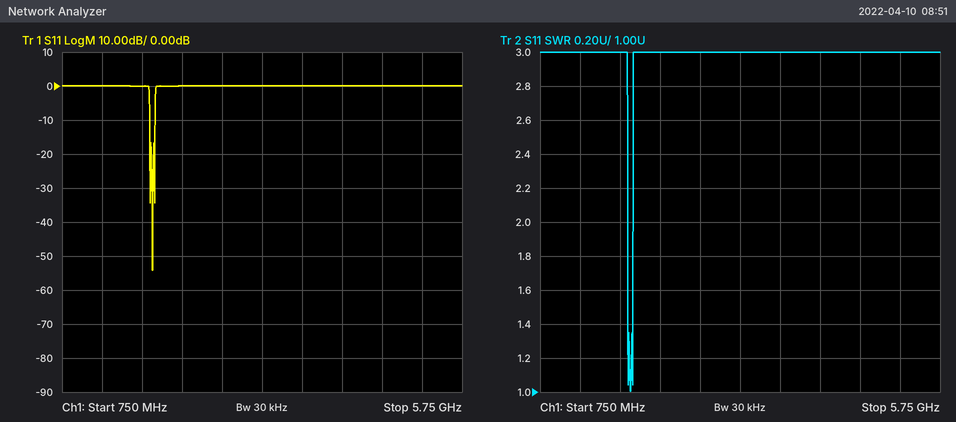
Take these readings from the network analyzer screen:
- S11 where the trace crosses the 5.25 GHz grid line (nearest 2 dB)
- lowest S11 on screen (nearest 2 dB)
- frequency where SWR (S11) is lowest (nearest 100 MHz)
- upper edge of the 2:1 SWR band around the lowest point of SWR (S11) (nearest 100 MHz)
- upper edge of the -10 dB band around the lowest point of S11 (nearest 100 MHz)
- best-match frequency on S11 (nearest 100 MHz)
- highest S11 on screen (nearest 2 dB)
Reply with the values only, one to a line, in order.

0 dB
-54 dB
1.9 GHz
1.9 GHz
1.9 GHz
1.9 GHz
0 dB
